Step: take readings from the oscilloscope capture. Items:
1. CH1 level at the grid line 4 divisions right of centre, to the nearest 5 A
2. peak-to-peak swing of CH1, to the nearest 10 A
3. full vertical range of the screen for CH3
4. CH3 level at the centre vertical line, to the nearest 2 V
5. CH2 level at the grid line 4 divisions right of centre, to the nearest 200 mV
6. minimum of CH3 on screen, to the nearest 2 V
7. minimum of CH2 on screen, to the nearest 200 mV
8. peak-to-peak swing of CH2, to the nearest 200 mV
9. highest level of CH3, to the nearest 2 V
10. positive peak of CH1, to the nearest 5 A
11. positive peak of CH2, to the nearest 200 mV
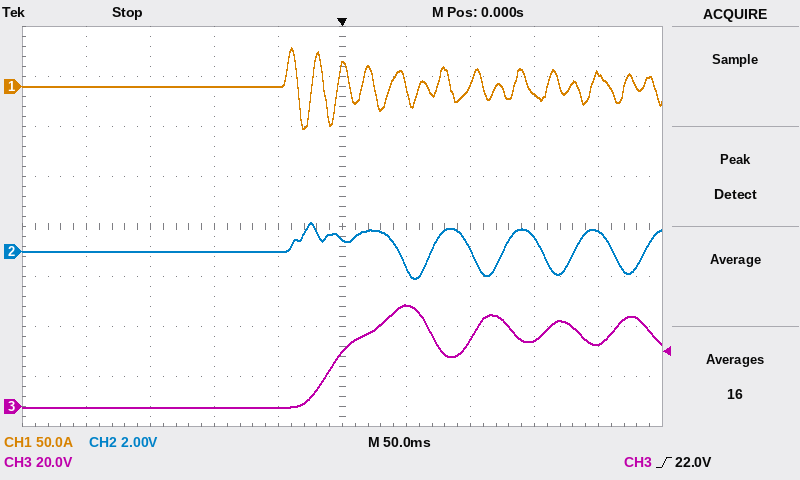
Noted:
15 A
80 A
160 V
22 V
800 mV
0 V
-1.0 V
2.2 V
40 V
40 A
1.2 V
